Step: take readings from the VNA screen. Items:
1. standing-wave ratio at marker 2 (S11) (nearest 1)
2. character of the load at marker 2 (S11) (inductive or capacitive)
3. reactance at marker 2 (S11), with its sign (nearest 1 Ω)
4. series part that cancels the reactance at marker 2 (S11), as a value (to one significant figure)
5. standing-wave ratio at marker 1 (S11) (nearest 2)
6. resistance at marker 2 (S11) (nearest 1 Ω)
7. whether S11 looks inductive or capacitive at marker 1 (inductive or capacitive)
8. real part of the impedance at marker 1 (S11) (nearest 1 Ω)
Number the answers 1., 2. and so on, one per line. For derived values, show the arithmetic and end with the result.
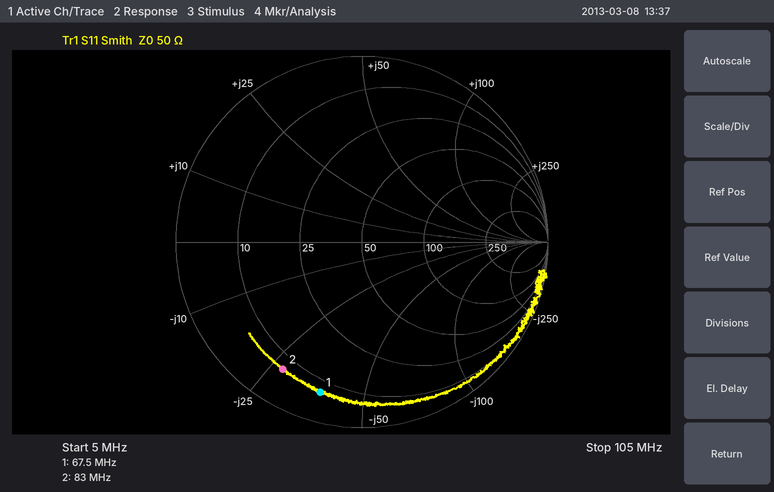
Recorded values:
1. 9
2. capacitive
3. -27 Ω
4. L = 27 Ω/(2π × 83 MHz) ≈ 51.8 nH, so 50 nH to one significant figure
5. 12
6. 7 Ω
7. capacitive
8. 7 Ω
